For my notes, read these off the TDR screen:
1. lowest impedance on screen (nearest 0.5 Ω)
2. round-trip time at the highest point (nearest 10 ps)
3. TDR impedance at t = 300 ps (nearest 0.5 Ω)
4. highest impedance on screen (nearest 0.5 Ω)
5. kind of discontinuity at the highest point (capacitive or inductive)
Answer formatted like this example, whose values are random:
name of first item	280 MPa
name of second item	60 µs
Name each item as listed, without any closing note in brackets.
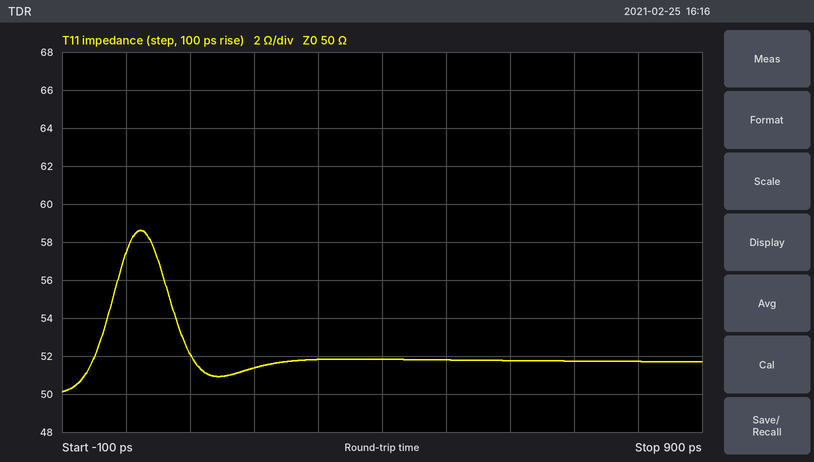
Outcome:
lowest impedance on screen	50.0 Ω
round-trip time at the highest point	20 ps
TDR impedance at t = 300 ps	52.0 Ω
highest impedance on screen	58.5 Ω
kind of discontinuity at the highest point	inductive
